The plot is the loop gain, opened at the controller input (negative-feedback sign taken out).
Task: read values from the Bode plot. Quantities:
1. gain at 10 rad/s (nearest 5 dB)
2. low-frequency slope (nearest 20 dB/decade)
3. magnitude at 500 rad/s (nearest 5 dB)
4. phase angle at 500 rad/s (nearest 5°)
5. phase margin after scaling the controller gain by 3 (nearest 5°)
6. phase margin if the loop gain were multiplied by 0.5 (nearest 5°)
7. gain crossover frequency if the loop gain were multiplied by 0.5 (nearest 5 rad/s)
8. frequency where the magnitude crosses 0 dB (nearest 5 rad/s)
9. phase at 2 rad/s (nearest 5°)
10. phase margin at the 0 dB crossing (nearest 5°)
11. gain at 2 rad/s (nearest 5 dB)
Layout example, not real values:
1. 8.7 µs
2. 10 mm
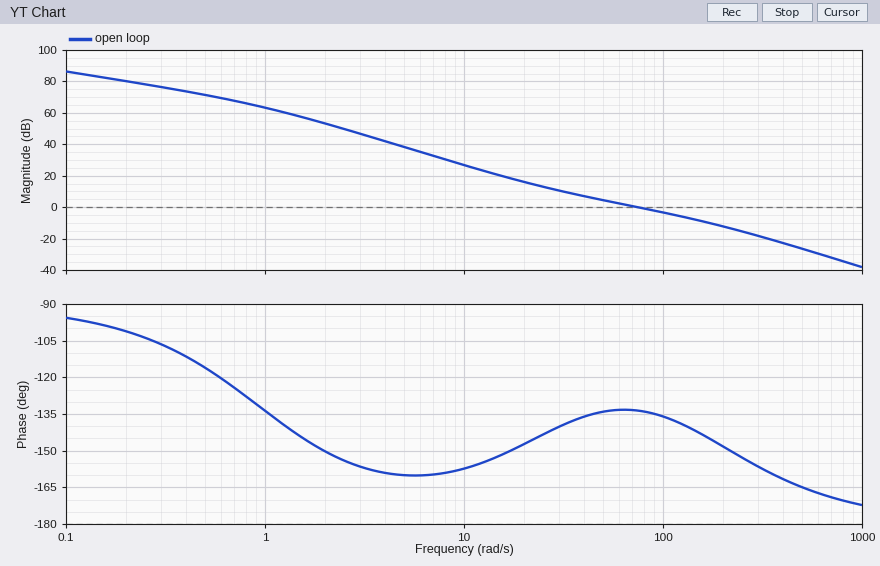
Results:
1. 25 dB
2. -20 dB/decade
3. -25 dB
4. -165°
5. 35°
6. 45°
7. 45 rad/s
8. 75 rad/s
9. -150°
10. 45°
11. 55 dB
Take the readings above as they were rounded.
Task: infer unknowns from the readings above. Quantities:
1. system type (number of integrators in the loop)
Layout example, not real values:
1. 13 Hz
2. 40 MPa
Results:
1. 1
